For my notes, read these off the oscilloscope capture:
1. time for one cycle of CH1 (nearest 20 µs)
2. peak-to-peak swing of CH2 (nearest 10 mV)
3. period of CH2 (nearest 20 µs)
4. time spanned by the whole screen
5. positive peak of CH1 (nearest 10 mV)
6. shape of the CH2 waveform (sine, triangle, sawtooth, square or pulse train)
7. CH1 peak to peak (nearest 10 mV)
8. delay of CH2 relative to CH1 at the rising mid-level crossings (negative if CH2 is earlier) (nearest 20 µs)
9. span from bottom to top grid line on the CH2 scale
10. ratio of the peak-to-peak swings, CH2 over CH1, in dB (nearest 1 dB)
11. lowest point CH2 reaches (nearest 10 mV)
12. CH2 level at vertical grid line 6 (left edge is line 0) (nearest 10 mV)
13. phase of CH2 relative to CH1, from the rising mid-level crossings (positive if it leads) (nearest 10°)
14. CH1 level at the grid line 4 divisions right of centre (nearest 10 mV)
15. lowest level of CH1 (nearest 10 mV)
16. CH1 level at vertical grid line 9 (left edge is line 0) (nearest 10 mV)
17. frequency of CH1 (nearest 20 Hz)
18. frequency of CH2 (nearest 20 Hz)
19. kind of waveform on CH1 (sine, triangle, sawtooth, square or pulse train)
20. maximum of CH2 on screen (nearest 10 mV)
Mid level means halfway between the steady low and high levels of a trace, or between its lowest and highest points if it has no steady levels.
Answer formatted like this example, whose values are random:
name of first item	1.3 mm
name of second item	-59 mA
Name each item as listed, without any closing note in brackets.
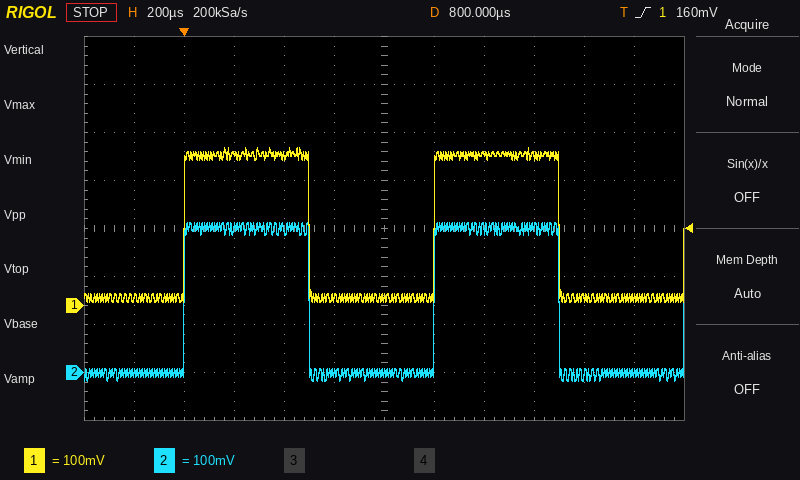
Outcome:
time for one cycle of CH1	1.00 ms
peak-to-peak swing of CH2	330 mV
period of CH2	1.00 ms
time spanned by the whole screen	2.4 ms
positive peak of CH1	330 mV
shape of the CH2 waveform	square
CH1 peak to peak	320 mV
delay of CH2 relative to CH1 at the rising mid-level crossings (negative if CH2 is earlier)	0 µs
span from bottom to top grid line on the CH2 scale	800 mV
ratio of the peak-to-peak swings, CH2 over CH1, in dB	0 dB
lowest point CH2 reaches	-20 mV
CH2 level at vertical grid line 6 (left edge is line 0)	0 mV
phase of CH2 relative to CH1, from the rising mid-level crossings (positive if it leads)	0°
CH1 level at the grid line 4 divisions right of centre	20 mV
lowest level of CH1	10 mV
CH1 level at vertical grid line 9 (left edge is line 0)	310 mV
frequency of CH1	1.00 kHz
frequency of CH2	1.00 kHz
kind of waveform on CH1	square
maximum of CH2 on screen	310 mV
